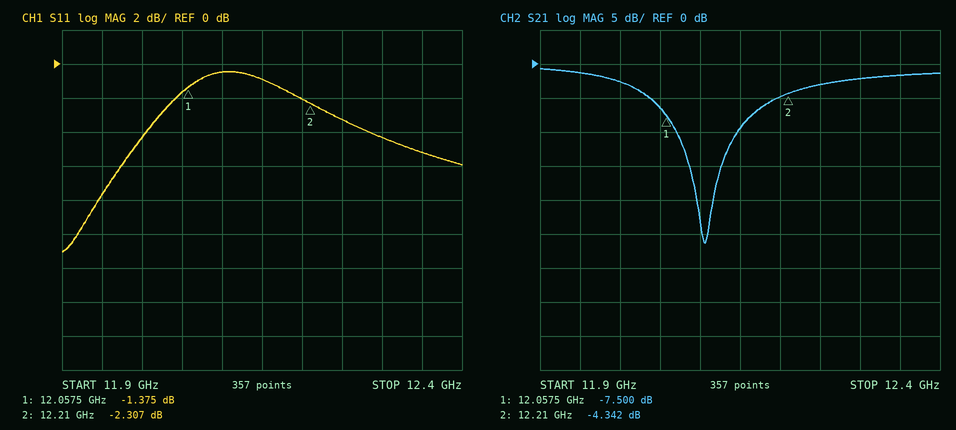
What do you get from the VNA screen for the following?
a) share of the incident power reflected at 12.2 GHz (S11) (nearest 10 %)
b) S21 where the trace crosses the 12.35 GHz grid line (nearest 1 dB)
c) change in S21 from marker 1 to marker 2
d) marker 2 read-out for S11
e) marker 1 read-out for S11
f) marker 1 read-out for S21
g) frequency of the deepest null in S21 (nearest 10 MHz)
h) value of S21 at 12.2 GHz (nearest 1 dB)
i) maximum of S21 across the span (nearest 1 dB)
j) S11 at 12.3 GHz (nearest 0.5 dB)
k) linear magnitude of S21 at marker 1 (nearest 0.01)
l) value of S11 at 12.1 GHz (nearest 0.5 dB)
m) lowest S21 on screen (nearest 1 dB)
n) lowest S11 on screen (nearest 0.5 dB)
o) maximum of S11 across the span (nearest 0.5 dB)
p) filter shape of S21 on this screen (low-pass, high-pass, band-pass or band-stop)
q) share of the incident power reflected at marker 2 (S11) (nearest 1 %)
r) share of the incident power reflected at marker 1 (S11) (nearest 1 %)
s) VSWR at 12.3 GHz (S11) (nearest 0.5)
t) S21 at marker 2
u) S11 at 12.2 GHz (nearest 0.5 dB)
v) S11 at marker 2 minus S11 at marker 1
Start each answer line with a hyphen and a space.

- 60 %
- -2 dB
- 3.158 dB
- -2.307 dB
- -1.375 dB
- -7.500 dB
- 12.11 GHz
- -5 dB
- -1 dB
- -4.5 dB
- 0.42
- -0.5 dB
- -26 dB
- -11.0 dB
- -0.5 dB
- band-stop
- 59 %
- 73 %
- 4.0
- -4.342 dB
- -2.0 dB
- -0.932 dB
